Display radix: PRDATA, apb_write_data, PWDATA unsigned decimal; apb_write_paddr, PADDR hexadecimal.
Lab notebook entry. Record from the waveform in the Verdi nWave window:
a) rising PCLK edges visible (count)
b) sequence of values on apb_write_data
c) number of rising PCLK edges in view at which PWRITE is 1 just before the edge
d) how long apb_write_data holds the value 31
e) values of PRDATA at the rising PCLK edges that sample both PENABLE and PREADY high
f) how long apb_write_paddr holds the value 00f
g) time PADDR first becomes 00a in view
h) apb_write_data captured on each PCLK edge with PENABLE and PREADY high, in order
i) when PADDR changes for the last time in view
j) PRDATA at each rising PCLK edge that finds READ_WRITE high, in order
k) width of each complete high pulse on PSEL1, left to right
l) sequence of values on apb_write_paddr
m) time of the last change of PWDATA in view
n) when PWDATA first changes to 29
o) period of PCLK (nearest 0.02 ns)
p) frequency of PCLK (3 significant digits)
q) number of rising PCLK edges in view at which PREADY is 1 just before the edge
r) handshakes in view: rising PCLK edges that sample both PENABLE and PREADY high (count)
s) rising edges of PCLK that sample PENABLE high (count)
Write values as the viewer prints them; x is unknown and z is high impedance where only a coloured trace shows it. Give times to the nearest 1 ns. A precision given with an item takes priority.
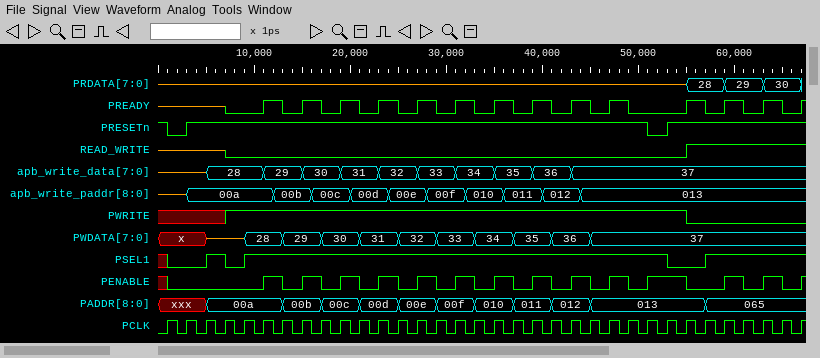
34
z, 28, 29, 30, 31, 32, 33, 34, 35, 36, 37
24
4 ns
z, z, z, z, z, z, z, z, z, z, 29, 30
4 ns
5 ns
29, 30, 31, 32, 33, 34, 35, 36, 37, 37, 37, 37
57 ns
28, 28, 29, 29, 30, 30
2 ns, 44 ns
z, 00a, 00b, 00c, 00d, 00e, 00f, 010, 011, 012, 013
45 ns
13 ns
2 ns
500 MHz
13
12
14
